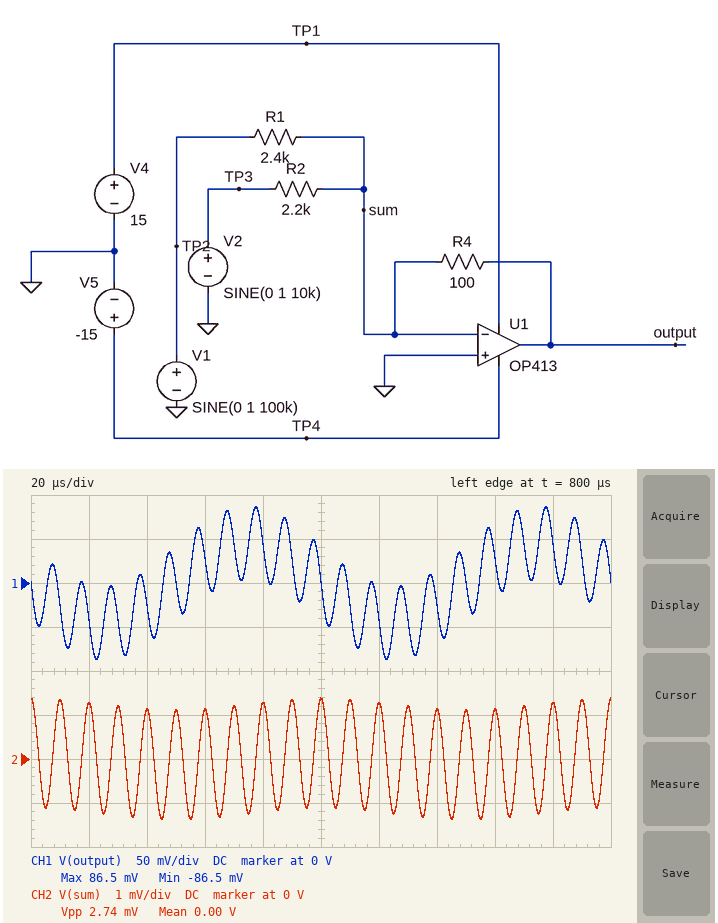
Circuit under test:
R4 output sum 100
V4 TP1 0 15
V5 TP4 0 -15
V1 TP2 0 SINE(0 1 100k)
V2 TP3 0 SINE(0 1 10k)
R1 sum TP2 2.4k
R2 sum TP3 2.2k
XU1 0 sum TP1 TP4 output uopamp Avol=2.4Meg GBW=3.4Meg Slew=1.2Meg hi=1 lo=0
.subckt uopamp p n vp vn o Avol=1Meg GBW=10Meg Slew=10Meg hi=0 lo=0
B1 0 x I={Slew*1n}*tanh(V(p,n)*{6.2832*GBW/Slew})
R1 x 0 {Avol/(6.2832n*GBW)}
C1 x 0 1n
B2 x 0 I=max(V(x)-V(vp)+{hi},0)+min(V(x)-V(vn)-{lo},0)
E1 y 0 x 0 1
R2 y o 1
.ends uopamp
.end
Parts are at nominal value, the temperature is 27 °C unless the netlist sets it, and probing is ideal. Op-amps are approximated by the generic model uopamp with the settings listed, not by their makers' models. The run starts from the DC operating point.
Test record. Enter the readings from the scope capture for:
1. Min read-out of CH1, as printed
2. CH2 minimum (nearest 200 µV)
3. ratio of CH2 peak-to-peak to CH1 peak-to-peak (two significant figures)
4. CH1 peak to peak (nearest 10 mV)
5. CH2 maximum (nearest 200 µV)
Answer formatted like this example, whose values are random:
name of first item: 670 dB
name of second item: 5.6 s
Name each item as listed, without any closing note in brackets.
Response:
Min read-out of CH1, as printed: -86.5 mV
CH2 minimum: -1.4 mV
ratio of CH2 peak-to-peak to CH1 peak-to-peak: 0.016
CH1 peak to peak: 170 mV
CH2 maximum: 1.4 mV
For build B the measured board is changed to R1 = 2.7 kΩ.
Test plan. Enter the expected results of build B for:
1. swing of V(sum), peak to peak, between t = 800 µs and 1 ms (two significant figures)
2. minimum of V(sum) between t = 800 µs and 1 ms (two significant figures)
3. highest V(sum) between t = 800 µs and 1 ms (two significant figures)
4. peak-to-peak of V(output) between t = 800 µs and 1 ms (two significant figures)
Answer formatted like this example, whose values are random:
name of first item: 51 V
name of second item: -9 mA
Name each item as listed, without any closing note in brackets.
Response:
swing of V(sum), peak to peak, between t = 800 µs and 1 ms: 2.5 mV
minimum of V(sum) between t = 800 µs and 1 ms: -1.2 mV
highest V(sum) between t = 800 µs and 1 ms: 1.2 mV
peak-to-peak of V(output) between t = 800 µs and 1 ms: 160 mV
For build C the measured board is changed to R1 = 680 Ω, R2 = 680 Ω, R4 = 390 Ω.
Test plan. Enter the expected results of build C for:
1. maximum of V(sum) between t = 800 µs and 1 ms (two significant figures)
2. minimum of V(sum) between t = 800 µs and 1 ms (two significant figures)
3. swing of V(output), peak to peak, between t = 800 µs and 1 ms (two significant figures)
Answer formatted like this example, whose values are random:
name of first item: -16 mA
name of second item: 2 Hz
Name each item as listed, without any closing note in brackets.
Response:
maximum of V(sum) between t = 800 µs and 1 ms: 19 mV
minimum of V(sum) between t = 800 µs and 1 ms: -19 mV
swing of V(output), peak to peak, between t = 800 µs and 1 ms: 2.3 V
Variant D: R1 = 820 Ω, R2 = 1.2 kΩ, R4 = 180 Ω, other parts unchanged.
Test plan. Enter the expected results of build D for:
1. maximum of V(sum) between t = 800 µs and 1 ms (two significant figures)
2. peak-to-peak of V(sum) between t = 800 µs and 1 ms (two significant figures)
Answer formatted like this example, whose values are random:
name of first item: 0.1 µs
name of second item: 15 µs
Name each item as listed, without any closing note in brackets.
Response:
maximum of V(sum) between t = 800 µs and 1 ms: 7.0 mV
peak-to-peak of V(sum) between t = 800 µs and 1 ms: 14 mV
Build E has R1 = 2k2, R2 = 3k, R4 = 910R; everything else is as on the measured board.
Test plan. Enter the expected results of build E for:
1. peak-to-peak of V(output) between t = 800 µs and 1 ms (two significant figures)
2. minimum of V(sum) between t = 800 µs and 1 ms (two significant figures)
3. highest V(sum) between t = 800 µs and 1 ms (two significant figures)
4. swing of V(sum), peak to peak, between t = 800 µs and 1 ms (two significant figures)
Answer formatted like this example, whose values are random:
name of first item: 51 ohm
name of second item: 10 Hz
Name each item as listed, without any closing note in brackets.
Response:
peak-to-peak of V(output) between t = 800 µs and 1 ms: 1.4 V
minimum of V(sum) between t = 800 µs and 1 ms: -13 mV
highest V(sum) between t = 800 µs and 1 ms: 13 mV
swing of V(sum), peak to peak, between t = 800 µs and 1 ms: 27 mV
